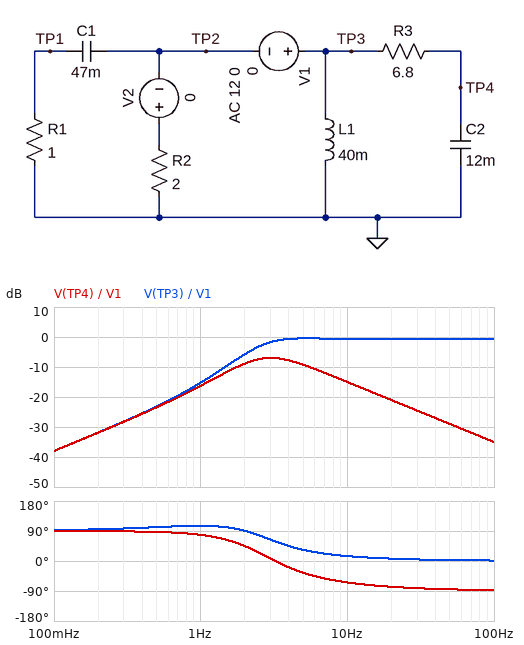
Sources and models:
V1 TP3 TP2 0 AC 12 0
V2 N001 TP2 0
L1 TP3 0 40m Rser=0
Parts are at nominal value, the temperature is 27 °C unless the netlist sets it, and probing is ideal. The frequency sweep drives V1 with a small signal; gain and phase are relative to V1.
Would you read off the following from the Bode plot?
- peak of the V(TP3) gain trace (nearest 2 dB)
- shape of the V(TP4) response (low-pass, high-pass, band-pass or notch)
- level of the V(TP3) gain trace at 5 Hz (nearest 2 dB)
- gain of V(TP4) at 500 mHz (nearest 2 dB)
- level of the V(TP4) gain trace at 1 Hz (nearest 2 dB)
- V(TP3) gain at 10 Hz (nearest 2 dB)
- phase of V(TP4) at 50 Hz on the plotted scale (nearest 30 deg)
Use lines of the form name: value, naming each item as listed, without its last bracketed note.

peak of the V(TP3) gain trace: 0 dB
shape of the V(TP4) response: band-pass
level of the V(TP3) gain trace at 5 Hz: 0 dB
gain of V(TP4) at 500 mHz: -24 dB
level of the V(TP4) gain trace at 1 Hz: -16 dB
V(TP3) gain at 10 Hz: 0 dB
phase of V(TP4) at 50 Hz on the plotted scale: -90 deg
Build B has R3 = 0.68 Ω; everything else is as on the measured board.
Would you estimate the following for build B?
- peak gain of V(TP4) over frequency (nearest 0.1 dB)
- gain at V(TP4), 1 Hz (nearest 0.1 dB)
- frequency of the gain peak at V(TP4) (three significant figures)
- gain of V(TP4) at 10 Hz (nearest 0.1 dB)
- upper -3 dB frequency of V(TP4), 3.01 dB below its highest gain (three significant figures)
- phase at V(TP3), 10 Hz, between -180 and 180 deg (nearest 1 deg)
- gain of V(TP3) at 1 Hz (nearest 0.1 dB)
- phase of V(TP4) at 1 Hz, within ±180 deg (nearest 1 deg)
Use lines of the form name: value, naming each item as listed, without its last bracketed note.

peak gain of V(TP4) over frequency: 0 dB
gain at V(TP4), 1 Hz: -15.2 dB
frequency of the gain peak at V(TP4): 3.96 Hz
gain of V(TP4) at 10 Hz: -2.9 dB
upper -3 dB frequency of V(TP4), 3.01 dB below its highest gain: 10.2 Hz
phase at V(TP3), 10 Hz, between -180 and 180 deg: -4 deg
gain of V(TP3) at 1 Hz: -15.2 dB
phase of V(TP4) at 1 Hz, within ±180 deg: 103 deg
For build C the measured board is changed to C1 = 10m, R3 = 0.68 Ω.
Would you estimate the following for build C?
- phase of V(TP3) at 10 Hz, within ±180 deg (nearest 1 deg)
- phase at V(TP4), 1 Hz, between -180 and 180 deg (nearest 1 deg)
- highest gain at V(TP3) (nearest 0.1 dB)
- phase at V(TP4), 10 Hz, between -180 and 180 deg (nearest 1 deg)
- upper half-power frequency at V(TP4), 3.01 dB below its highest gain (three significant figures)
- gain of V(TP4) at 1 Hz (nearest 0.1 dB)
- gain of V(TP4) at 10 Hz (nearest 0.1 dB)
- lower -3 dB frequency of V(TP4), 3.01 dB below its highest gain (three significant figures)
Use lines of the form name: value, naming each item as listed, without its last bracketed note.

phase of V(TP3) at 10 Hz, within ±180 deg: -1 deg
phase at V(TP4), 1 Hz, between -180 and 180 deg: 87 deg
highest gain at V(TP3): -0.4 dB
phase at V(TP4), 10 Hz, between -180 and 180 deg: -28 deg
upper half-power frequency at V(TP4), 3.01 dB below its highest gain: 9.67 Hz
gain of V(TP4) at 1 Hz: -17.7 dB
gain of V(TP4) at 10 Hz: -4.0 dB
lower -3 dB frequency of V(TP4), 3.01 dB below its highest gain: 3.52 Hz
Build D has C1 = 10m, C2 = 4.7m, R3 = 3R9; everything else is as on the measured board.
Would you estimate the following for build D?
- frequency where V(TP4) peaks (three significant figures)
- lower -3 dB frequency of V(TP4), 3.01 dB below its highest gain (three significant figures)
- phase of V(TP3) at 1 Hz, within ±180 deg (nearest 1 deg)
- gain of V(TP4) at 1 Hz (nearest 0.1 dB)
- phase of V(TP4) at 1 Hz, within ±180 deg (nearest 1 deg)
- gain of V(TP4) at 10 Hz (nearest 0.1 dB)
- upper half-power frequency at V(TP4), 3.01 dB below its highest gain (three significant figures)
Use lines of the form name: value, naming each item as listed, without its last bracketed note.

frequency where V(TP4) peaks: 6.13 Hz
lower -3 dB frequency of V(TP4), 3.01 dB below its highest gain: 3.64 Hz
phase of V(TP3) at 1 Hz, within ±180 deg: 90 deg
gain of V(TP4) at 1 Hz: -17.8 dB
phase of V(TP4) at 1 Hz, within ±180 deg: 83 deg
gain of V(TP4) at 10 Hz: -4.1 dB
upper half-power frequency at V(TP4), 3.01 dB below its highest gain: 11.6 Hz
